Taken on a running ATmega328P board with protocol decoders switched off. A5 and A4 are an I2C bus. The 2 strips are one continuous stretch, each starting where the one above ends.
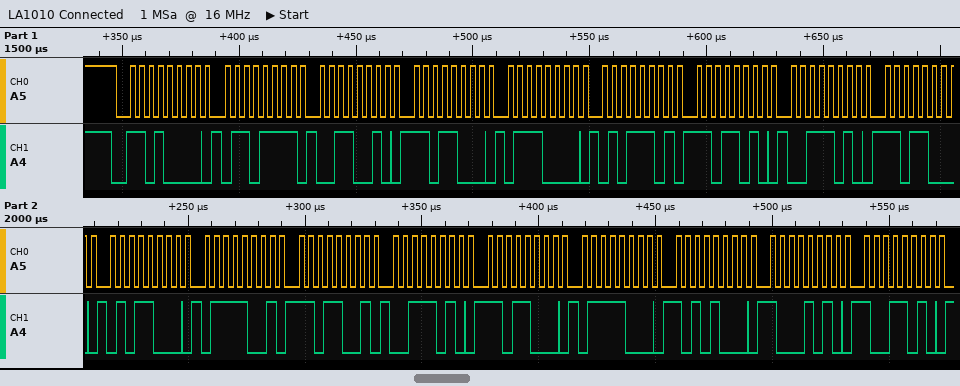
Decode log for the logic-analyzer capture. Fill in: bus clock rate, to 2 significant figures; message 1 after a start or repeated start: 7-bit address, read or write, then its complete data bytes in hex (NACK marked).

250 kHz
0x68 write: 6F 32 D8 70 5D DA 3A D8 58 79 D9 3A D8 78 A8 8A 9A
